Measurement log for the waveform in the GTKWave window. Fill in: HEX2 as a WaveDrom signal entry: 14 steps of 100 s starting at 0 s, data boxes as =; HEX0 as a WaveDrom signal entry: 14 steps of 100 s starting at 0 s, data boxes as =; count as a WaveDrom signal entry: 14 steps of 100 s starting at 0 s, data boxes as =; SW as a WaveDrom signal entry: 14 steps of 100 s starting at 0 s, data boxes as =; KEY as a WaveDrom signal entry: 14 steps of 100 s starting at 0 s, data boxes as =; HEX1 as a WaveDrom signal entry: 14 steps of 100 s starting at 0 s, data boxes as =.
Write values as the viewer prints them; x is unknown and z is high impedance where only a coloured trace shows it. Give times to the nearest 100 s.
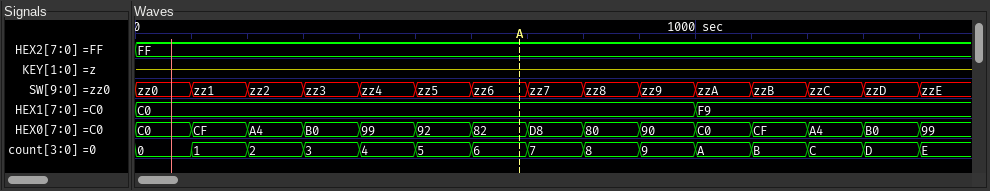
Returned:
{name: 'HEX2', wave: '=.............', data: 'FF'}
{name: 'HEX0', wave: '==============', data: 'C0 CF A4 B0 99 92 82 D8 80 90 C0 CF A4 B0'}
{name: 'count', wave: '==============', data: '0 1 2 3 4 5 6 7 8 9 A B C D'}
{name: 'SW', wave: '==============', data: 'zz0 zz1 zz2 zz3 zz4 zz5 zz6 zz7 zz8 zz9 zzA zzB zzC zzD'}
{name: 'KEY', wave: 'z.............'}
{name: 'HEX1', wave: '=.........=...', data: 'C0 F9'}
